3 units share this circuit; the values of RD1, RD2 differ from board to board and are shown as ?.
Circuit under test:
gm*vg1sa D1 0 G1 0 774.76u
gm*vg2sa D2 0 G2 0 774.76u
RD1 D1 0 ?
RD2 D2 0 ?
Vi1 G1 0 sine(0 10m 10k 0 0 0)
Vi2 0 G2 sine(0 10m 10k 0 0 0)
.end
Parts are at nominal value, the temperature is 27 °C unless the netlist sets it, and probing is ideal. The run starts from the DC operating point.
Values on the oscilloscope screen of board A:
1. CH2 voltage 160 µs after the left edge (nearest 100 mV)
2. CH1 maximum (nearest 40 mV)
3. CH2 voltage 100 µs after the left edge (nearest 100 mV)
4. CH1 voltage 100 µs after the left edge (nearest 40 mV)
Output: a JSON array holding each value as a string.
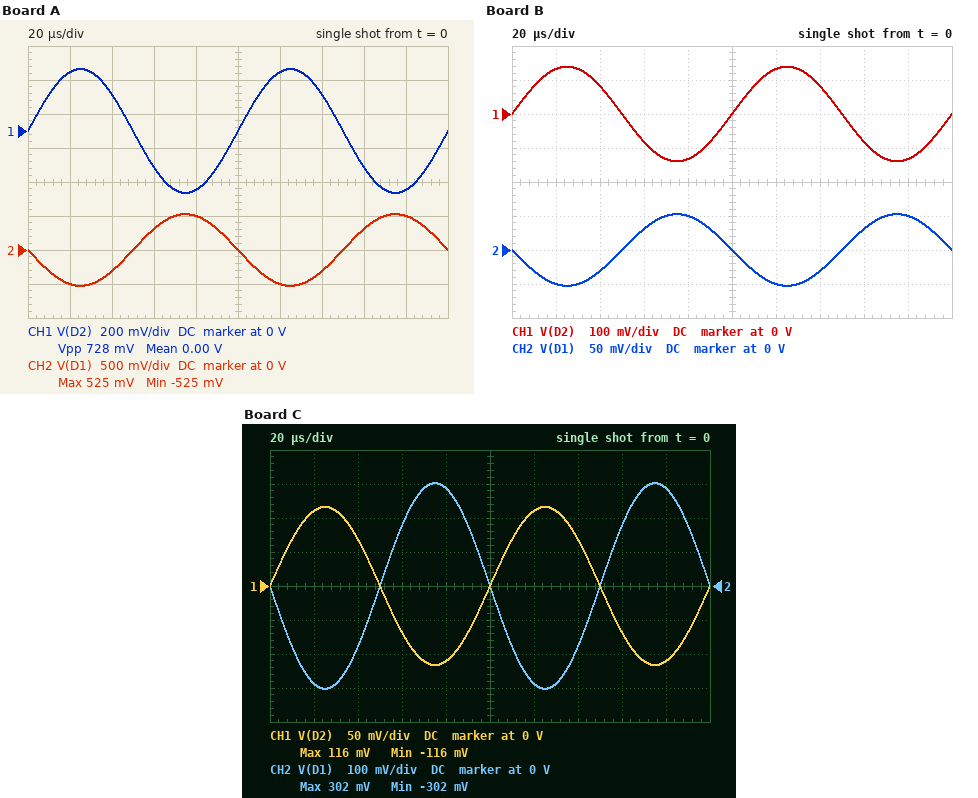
["300 mV", "360 mV", "0 V", "0 V"]
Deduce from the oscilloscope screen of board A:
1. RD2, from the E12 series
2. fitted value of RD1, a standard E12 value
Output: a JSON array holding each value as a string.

["47 kΩ", "68 kΩ"]
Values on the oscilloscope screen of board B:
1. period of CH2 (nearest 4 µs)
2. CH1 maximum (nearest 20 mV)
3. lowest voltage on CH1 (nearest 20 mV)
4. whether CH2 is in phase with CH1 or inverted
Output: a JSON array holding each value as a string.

["100 µs", "140 mV", "-140 mV", "inverted"]
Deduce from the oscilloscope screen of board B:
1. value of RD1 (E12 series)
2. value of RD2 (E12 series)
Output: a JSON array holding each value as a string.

["6.8 kΩ", "18 kΩ"]
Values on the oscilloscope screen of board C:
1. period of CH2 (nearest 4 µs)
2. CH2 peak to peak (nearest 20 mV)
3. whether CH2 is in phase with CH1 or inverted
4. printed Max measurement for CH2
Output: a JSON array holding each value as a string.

["100 µs", "600 mV", "inverted", "302 mV"]
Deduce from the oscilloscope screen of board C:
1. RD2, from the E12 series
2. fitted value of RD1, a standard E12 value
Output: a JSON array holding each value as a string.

["15 kΩ", "39 kΩ"]
